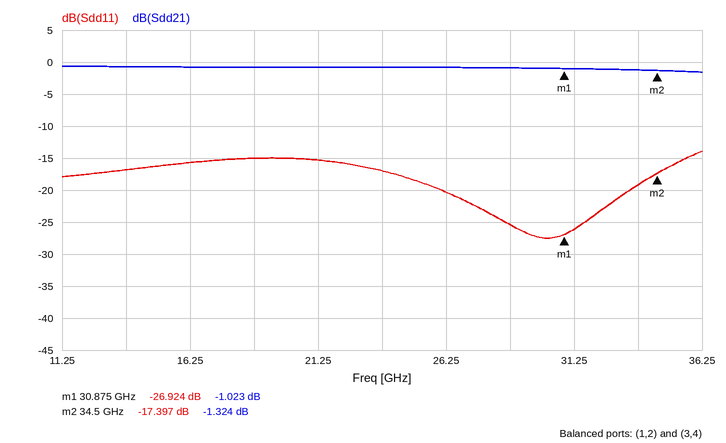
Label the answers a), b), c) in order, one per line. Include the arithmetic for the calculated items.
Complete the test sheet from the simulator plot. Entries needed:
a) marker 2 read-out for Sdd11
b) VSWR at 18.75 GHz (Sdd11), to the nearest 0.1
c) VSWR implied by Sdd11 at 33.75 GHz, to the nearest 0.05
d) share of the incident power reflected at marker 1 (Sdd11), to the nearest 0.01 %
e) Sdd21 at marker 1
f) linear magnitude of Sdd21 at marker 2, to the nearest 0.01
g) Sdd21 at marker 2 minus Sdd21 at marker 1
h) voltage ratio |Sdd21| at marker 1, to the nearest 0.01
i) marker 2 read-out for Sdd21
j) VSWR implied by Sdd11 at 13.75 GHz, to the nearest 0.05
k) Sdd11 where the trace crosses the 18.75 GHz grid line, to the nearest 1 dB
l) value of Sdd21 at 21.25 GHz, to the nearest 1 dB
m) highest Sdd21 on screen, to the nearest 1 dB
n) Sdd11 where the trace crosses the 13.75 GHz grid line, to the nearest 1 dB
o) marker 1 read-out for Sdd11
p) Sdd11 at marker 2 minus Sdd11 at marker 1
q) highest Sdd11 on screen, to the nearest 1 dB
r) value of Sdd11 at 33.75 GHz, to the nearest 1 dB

a) -17.397 dB
b) |Γ| = 10^(-15/20) = 0.1778; VSWR = (1 + 0.1778)/(1 − 0.1778) ≈ 1.4
c) |Γ| = 10^(-19/20) = 0.1122; VSWR = (1 + 0.1122)/(1 − 0.1122) ≈ 1.25
d) 10^(-26.924/10) ≈ 0.20 %
e) -1.023 dB
f) 10^(-1.324/20) ≈ 0.86
g) -1.324 − (-1.023) = -0.301 dB
h) 10^(-1.023/20) ≈ 0.89
i) -1.324 dB
j) |Γ| = 10^(-17/20) = 0.1413; VSWR = (1 + 0.1413)/(1 − 0.1413) ≈ 1.33, so 1.35 to the nearest 0.05
k) -15 dB
l) -1 dB
m) -1 dB
n) -17 dB
o) -26.924 dB
p) -17.397 − (-26.924) = 9.527 dB
q) -14 dB
r) -19 dB
